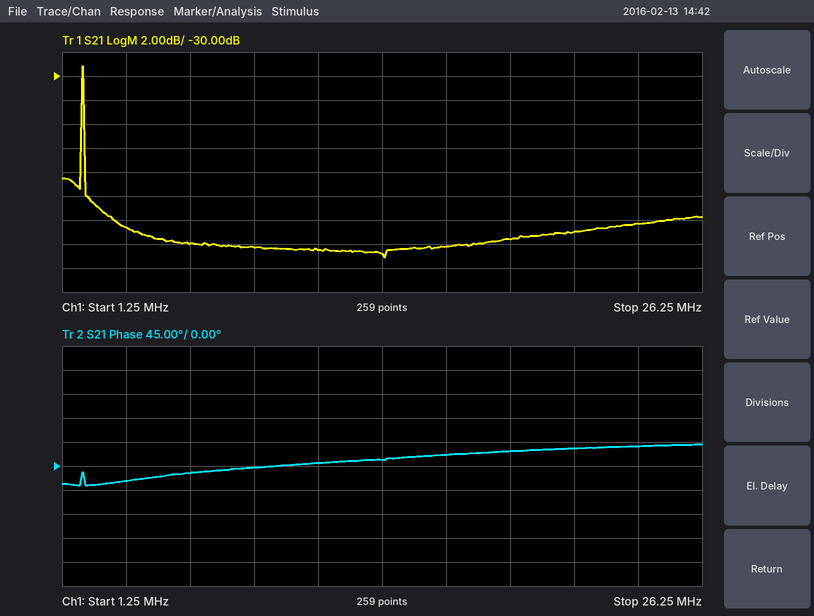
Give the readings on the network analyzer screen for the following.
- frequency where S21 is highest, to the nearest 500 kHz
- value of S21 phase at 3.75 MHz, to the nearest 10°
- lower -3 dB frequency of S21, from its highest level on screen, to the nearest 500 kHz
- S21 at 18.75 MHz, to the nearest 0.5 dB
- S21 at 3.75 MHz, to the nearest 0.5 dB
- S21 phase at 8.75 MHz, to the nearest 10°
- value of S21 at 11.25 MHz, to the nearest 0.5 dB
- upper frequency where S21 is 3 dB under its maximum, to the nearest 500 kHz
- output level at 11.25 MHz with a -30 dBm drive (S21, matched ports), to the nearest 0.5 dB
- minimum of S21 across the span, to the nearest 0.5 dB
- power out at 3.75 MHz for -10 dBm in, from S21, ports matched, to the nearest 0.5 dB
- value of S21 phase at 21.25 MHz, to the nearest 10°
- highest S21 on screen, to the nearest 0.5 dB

2.0 MHz
-30°
2.0 MHz
-43.5 dB
-42.5 dB
0°
-44.5 dB
2.0 MHz
-74.5 dBm
-45.0 dB
-52.5 dBm
30°
-29.0 dB
